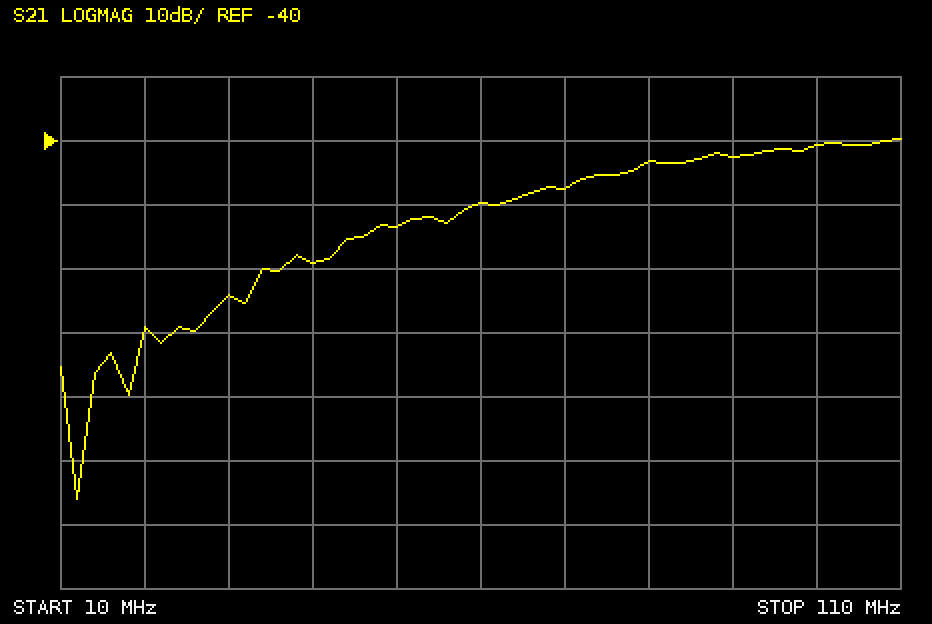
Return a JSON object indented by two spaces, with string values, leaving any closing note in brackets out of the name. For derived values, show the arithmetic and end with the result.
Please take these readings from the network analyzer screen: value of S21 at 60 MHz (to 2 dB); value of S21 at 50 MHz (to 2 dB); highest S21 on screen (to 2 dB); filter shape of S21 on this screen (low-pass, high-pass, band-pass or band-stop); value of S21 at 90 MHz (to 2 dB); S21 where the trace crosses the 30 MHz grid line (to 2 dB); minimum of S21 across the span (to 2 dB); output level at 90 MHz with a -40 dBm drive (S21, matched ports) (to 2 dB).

{
  "value of S21 at 60 MHz": "-50 dB",
  "value of S21 at 50 MHz": "-54 dB",
  "highest S21 on screen": "-40 dB",
  "filter shape of S21 on this screen": "high-pass",
  "value of S21 at 90 MHz": "-42 dB",
  "S21 where the trace crosses the 30 MHz grid line": "-64 dB",
  "minimum of S21 across the span": "-96 dB",
  "output level at 90 MHz with a -40 dBm drive (S21, matched ports)": "-40 dBm + (-42 dB) = -82 dBm"
}
